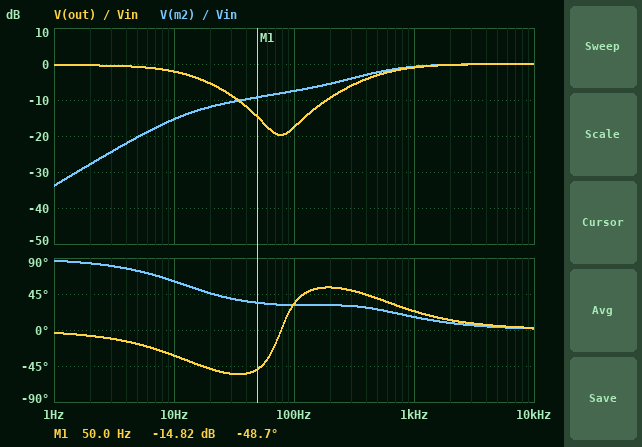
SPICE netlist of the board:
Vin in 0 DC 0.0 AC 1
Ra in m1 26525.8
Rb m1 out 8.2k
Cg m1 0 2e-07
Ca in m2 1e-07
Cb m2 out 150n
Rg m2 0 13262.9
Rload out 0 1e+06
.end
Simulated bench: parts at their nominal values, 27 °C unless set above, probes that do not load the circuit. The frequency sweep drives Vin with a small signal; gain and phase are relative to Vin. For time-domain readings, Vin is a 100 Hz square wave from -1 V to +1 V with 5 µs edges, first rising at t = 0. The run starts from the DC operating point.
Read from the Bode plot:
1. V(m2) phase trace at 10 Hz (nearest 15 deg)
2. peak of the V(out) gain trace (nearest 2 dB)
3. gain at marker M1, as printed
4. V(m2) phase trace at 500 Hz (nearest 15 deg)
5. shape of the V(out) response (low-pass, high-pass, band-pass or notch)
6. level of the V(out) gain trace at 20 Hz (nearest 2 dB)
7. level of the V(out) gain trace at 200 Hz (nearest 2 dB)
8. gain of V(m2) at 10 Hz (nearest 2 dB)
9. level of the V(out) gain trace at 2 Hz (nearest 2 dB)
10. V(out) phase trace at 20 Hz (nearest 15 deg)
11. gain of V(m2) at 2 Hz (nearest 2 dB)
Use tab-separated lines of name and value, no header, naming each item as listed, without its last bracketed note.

V(m2) phase trace at 10 Hz	60 deg
peak of the V(out) gain trace	0 dB
gain at marker M1, as printed	-14.82 dB
V(m2) phase trace at 500 Hz	30 deg
shape of the V(out) response	notch
level of the V(out) gain trace at 20 Hz	-6 dB
level of the V(out) gain trace at 200 Hz	-10 dB
gain of V(m2) at 10 Hz	-16 dB
level of the V(out) gain trace at 2 Hz	0 dB
V(out) phase trace at 20 Hz	-45 deg
gain of V(m2) at 2 Hz	-28 dB
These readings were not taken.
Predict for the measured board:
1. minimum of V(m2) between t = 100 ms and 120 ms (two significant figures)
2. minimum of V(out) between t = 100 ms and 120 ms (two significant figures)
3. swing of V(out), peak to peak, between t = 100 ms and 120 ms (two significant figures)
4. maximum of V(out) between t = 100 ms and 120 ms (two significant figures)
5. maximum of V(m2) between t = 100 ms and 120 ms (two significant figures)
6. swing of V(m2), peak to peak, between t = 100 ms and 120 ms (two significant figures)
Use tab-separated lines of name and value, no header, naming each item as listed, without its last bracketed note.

minimum of V(m2) between t = 100 ms and 120 ms	-1.8 V
minimum of V(out) between t = 100 ms and 120 ms	-1.7 V
swing of V(out), peak to peak, between t = 100 ms and 120 ms	3.5 V
maximum of V(out) between t = 100 ms and 120 ms	1.7 V
maximum of V(m2) between t = 100 ms and 120 ms	1.8 V
swing of V(m2), peak to peak, between t = 100 ms and 120 ms	3.5 V
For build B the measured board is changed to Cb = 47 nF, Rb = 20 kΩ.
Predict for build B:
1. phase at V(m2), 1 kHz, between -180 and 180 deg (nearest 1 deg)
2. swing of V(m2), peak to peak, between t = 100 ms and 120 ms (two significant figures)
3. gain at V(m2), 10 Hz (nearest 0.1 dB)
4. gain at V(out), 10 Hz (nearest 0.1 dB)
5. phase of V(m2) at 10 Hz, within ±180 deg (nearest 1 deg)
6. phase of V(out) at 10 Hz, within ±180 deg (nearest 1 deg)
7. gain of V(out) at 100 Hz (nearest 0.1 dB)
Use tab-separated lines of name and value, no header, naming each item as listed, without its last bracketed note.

phase at V(m2), 1 kHz, between -180 and 180 deg	11 deg
swing of V(m2), peak to peak, between t = 100 ms and 120 ms	3.7 V
gain at V(m2), 10 Hz	-18.8 dB
gain at V(out), 10 Hz	-1.2 dB
phase of V(m2) at 10 Hz, within ±180 deg	76 deg
phase of V(out) at 10 Hz, within ±180 deg	-25 deg
gain of V(out) at 100 Hz	-24.8 dB
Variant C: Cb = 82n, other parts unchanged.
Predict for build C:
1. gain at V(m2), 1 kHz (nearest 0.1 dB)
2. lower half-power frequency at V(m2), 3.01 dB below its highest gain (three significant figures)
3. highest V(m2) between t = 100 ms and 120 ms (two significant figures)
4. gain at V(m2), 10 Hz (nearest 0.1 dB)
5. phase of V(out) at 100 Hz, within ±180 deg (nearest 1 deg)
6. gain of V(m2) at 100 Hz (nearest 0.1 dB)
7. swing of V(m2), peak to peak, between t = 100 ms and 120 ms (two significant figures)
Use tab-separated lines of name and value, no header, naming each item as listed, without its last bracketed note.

gain at V(m2), 1 kHz	-0.9 dB
lower half-power frequency at V(m2), 3.01 dB below its highest gain	383 Hz
highest V(m2) between t = 100 ms and 120 ms	1.8 V
gain at V(m2), 10 Hz	-17.3 dB
phase of V(out) at 100 Hz, within ±180 deg	4 deg
gain of V(m2) at 100 Hz	-6.3 dB
swing of V(m2), peak to peak, between t = 100 ms and 120 ms	3.6 V
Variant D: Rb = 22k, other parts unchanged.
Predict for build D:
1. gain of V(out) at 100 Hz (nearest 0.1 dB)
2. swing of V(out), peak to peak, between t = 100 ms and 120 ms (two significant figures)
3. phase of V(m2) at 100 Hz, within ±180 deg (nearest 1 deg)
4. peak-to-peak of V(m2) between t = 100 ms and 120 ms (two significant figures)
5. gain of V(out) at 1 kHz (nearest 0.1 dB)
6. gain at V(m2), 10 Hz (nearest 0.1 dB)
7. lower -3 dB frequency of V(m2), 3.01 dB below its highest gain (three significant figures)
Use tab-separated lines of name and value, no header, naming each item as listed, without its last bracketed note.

gain of V(out) at 100 Hz	-11.5 dB
swing of V(out), peak to peak, between t = 100 ms and 120 ms	3.7 V
phase of V(m2) at 100 Hz, within ±180 deg	43 deg
peak-to-peak of V(m2) between t = 100 ms and 120 ms	3.6 V
gain of V(out) at 1 kHz	-0.3 dB
gain at V(m2), 10 Hz	-15.8 dB
lower -3 dB frequency of V(m2), 3.01 dB below its highest gain	228 Hz
